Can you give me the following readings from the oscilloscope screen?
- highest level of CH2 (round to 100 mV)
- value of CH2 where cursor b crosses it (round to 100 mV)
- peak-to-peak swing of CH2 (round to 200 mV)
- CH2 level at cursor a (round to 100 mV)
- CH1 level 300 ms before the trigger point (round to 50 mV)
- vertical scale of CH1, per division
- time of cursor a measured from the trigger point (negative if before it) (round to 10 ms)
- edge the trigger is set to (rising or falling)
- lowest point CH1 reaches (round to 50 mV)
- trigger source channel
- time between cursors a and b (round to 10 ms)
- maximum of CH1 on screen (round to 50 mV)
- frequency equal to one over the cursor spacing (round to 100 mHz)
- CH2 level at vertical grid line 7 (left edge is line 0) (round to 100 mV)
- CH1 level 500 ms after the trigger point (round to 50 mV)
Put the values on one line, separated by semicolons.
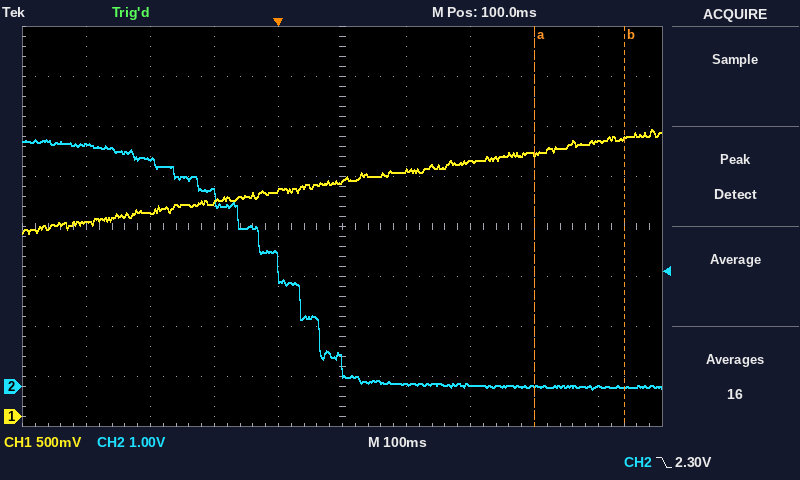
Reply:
4.9 V; 0.0 V; 5.0 V; 0.0 V; 1.95 V; 500 mV; +400 ms; falling; 1.85 V; CH2; 140 ms; 2.85 V; 7.1 Hz; 0.0 V; 2.75 V
